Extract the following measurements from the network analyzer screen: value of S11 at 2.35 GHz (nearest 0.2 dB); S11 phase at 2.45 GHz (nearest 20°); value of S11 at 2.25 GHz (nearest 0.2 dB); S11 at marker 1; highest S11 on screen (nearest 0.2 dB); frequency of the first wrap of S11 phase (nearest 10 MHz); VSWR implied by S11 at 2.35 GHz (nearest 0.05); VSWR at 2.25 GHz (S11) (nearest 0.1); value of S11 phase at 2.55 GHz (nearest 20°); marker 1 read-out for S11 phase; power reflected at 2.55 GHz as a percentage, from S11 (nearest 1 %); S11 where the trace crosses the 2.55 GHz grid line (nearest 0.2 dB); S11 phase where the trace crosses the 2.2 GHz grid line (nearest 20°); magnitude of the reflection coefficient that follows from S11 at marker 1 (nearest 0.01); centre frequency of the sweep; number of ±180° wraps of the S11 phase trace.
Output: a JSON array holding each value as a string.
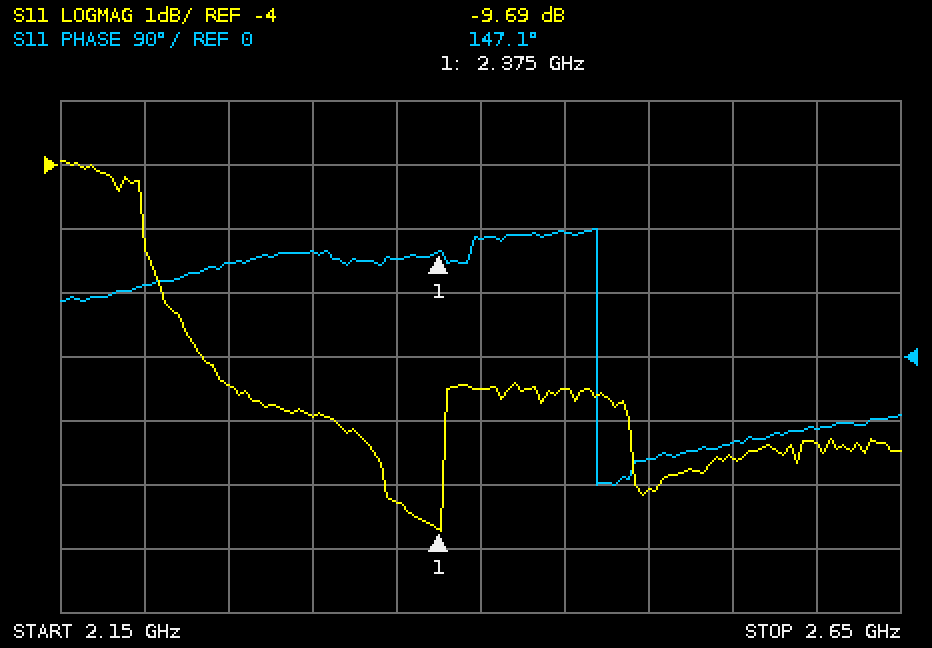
["-9.2 dB", "180°", "-7.4 dB", "-9.69 dB", "-4.0 dB", "2.47 GHz", "2.05", "2.5", "-120°", "147.1°", "14 %", "-8.6 dB", "100°", "0.33", "2.4 GHz", "1"]
